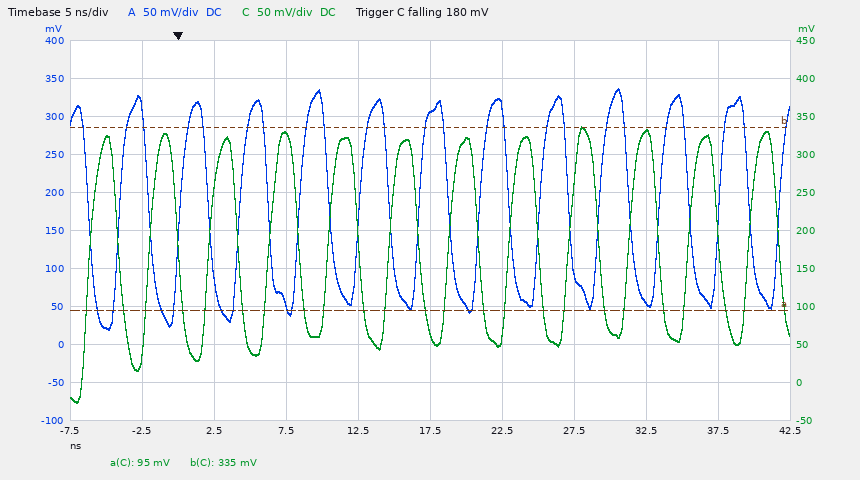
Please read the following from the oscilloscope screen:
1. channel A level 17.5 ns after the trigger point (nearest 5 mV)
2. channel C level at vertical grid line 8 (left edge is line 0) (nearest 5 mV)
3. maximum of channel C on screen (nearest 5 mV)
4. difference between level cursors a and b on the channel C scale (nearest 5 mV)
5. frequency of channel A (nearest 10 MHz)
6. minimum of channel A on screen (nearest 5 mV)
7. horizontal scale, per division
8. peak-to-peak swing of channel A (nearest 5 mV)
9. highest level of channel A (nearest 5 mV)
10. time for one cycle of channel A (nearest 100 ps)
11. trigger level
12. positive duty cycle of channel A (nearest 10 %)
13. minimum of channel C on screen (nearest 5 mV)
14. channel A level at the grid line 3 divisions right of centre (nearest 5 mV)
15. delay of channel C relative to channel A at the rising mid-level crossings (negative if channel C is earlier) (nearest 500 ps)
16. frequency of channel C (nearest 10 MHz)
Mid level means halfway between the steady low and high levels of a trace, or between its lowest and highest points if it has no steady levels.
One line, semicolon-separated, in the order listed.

305 mV; 330 mV; 335 mV; 240 mV; 240 MHz; 20 mV; 5 ns; 315 mV; 335 mV; 4.2 ns; 180 mV; 50 %; -25 mV; 55 mV; +2.0 ns; 240 MHz
